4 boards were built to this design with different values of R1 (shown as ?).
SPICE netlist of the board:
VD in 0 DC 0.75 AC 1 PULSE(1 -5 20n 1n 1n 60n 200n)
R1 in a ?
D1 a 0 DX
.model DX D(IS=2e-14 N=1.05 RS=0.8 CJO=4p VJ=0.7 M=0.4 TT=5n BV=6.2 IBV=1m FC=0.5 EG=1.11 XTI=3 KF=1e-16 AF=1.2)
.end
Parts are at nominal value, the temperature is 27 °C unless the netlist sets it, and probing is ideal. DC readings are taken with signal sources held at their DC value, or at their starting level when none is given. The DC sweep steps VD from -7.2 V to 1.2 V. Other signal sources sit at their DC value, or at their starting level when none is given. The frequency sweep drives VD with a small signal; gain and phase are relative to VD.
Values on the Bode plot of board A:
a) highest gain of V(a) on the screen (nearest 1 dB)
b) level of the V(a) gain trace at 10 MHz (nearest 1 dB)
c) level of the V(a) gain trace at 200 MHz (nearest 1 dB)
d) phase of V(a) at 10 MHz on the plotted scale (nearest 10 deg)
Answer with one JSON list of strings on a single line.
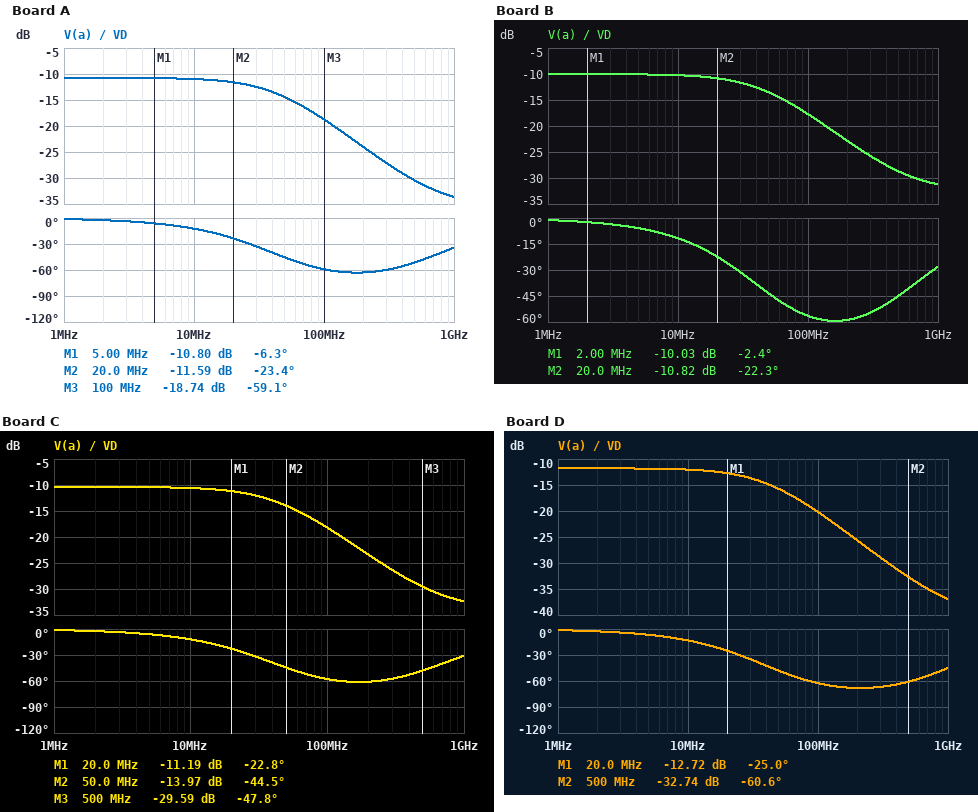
["-11 dB", "-11 dB", "-24 dB", "-10 deg"]
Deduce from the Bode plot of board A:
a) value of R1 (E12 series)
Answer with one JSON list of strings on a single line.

["47 Ω"]
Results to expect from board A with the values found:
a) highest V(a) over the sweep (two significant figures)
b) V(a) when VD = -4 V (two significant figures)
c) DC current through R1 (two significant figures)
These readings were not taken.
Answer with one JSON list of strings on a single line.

["740 mV", "-4.0 V", "1.5 mA"]
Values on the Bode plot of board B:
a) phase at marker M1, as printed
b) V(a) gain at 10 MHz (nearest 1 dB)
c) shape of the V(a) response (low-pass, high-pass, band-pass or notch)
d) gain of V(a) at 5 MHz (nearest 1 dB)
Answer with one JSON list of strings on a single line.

["-2.4 deg", "-10 dB", "low-pass", "-10 dB"]
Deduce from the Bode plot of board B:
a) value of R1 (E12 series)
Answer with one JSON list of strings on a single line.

["33 Ω"]
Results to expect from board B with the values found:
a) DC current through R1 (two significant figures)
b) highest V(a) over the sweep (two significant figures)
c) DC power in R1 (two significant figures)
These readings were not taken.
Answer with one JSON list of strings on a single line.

["1.9 mA", "750 mV", "120 µW"]
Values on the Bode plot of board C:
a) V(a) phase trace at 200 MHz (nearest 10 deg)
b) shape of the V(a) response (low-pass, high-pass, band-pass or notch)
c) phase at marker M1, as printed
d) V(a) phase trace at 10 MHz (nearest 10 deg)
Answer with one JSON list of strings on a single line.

["-60 deg", "low-pass", "-22.8 deg", "-10 deg"]
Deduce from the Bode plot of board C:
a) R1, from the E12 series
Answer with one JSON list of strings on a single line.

["39 Ω"]
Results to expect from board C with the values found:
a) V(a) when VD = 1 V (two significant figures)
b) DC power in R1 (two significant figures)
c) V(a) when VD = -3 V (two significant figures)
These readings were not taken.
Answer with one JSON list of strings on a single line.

["730 mV", "110 µW", "-3.0 V"]
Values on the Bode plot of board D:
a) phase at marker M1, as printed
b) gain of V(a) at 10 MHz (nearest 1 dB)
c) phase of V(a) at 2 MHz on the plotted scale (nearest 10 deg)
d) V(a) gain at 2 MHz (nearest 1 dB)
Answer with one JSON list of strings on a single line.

["-25.0 deg", "-12 dB", "0 deg", "-12 dB"]
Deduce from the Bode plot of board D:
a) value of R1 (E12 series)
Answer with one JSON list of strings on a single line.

["82 Ω"]
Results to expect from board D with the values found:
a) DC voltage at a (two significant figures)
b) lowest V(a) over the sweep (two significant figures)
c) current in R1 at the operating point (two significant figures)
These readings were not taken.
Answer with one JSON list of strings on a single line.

["670 mV", "-6.3 V", "980 µA"]
